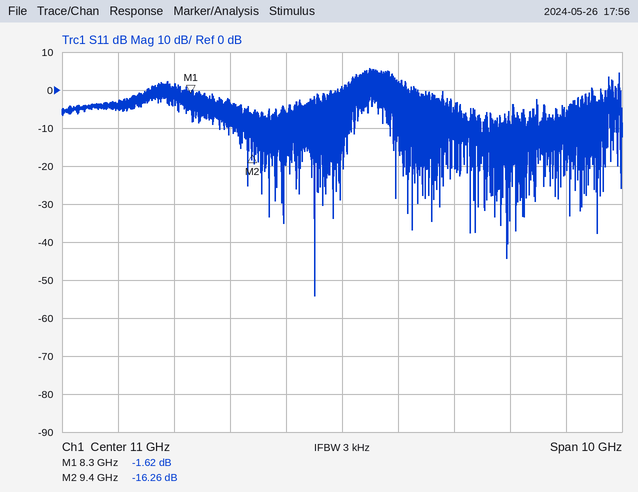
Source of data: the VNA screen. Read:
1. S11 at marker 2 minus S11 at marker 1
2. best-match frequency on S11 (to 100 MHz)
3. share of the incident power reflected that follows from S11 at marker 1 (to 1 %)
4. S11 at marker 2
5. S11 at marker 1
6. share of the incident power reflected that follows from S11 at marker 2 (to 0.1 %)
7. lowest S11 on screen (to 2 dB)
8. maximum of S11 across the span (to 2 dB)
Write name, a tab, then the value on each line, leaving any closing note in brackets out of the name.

S11 at marker 2 minus S11 at marker 1	-14.64 dB
best-match frequency on S11	10.5 GHz
share of the incident power reflected that follows from S11 at marker 1	69 %
S11 at marker 2	-16.26 dB
S11 at marker 1	-1.62 dB
share of the incident power reflected that follows from S11 at marker 2	2.4 %
lowest S11 on screen	-54 dB
maximum of S11 across the span	6 dB
